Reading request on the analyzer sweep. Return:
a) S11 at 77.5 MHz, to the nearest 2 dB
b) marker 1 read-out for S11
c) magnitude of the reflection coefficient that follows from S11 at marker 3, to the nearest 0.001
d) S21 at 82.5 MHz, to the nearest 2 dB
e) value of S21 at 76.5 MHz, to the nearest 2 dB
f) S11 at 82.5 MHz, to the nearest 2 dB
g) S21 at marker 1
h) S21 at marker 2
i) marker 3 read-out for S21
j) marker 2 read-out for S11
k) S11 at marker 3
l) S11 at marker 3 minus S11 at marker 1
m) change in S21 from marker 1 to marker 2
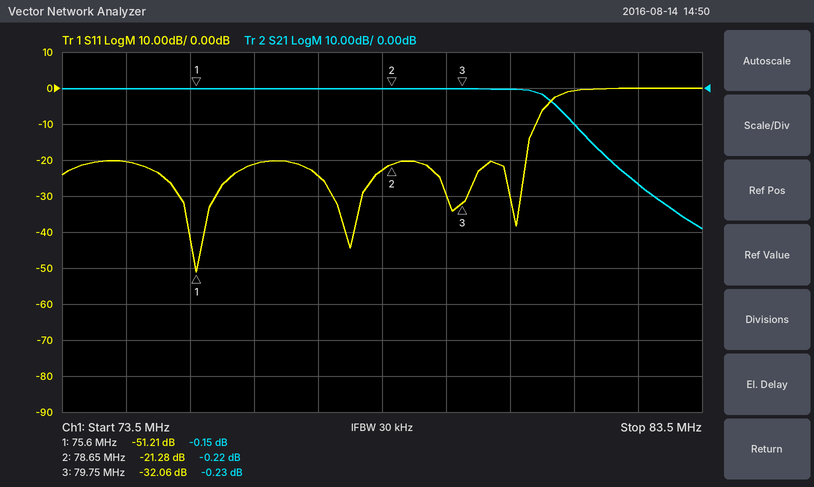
-24 dB
-51.21 dB
0.025
-26 dB
0 dB
0 dB
-0.15 dB
-0.22 dB
-0.23 dB
-21.28 dB
-32.06 dB
19.15 dB
-0.07 dB
